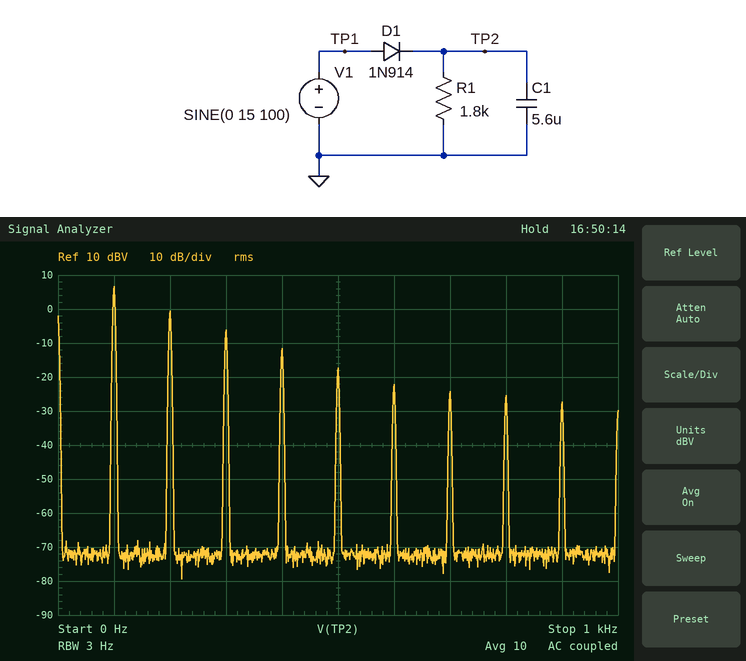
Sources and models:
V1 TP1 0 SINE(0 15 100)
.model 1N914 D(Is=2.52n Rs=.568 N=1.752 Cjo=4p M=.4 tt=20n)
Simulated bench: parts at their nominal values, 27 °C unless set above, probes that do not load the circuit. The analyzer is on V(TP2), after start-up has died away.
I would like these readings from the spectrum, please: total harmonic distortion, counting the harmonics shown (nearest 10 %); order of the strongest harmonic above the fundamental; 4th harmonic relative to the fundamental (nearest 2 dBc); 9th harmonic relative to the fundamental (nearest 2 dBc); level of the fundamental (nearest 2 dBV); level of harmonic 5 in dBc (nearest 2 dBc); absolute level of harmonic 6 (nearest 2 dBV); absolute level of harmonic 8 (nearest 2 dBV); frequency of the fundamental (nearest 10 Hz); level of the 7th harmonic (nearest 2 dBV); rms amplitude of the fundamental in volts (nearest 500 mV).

50 %
2
-18 dBc
-34 dBc
6 dBV
-24 dBc
-22 dBV
-26 dBV
100 Hz
-24 dBV
2.0 V
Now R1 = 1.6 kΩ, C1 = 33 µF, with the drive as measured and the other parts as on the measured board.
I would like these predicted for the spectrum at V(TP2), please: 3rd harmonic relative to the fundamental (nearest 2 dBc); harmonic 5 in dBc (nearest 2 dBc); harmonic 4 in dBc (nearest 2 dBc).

-10 dBc
-16 dBc
-14 dBc
